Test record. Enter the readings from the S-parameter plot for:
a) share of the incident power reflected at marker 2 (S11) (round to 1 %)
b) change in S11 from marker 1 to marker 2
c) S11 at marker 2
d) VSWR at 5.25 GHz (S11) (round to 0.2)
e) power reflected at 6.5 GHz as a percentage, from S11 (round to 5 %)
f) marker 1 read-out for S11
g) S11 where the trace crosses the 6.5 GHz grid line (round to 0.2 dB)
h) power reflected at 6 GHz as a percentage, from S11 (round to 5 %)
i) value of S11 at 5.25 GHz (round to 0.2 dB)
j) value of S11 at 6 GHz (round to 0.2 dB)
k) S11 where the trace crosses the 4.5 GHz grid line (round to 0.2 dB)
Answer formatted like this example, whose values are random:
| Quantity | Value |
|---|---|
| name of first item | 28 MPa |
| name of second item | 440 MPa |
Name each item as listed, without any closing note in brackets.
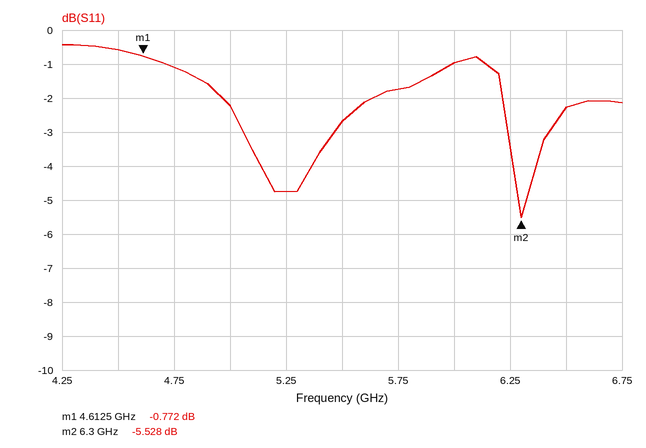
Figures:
| Quantity | Value |
|---|---|
| share of the incident power reflected at marker 2 (S11) | 28 % |
| change in S11 from marker 1 to marker 2 | -4.756 dB |
| S11 at marker 2 | -5.528 dB |
| VSWR at 5.25 GHz (S11) | 3.8 |
| power reflected at 6.5 GHz as a percentage, from S11 | 60 % |
| marker 1 read-out for S11 | -0.772 dB |
| S11 where the trace crosses the 6.5 GHz grid line | -2.2 dB |
| power reflected at 6 GHz as a percentage, from S11 | 80 % |
| value of S11 at 5.25 GHz | -4.8 dB |
| value of S11 at 6 GHz | -1.0 dB |
| S11 where the trace crosses the 4.5 GHz grid line | -0.6 dB |
